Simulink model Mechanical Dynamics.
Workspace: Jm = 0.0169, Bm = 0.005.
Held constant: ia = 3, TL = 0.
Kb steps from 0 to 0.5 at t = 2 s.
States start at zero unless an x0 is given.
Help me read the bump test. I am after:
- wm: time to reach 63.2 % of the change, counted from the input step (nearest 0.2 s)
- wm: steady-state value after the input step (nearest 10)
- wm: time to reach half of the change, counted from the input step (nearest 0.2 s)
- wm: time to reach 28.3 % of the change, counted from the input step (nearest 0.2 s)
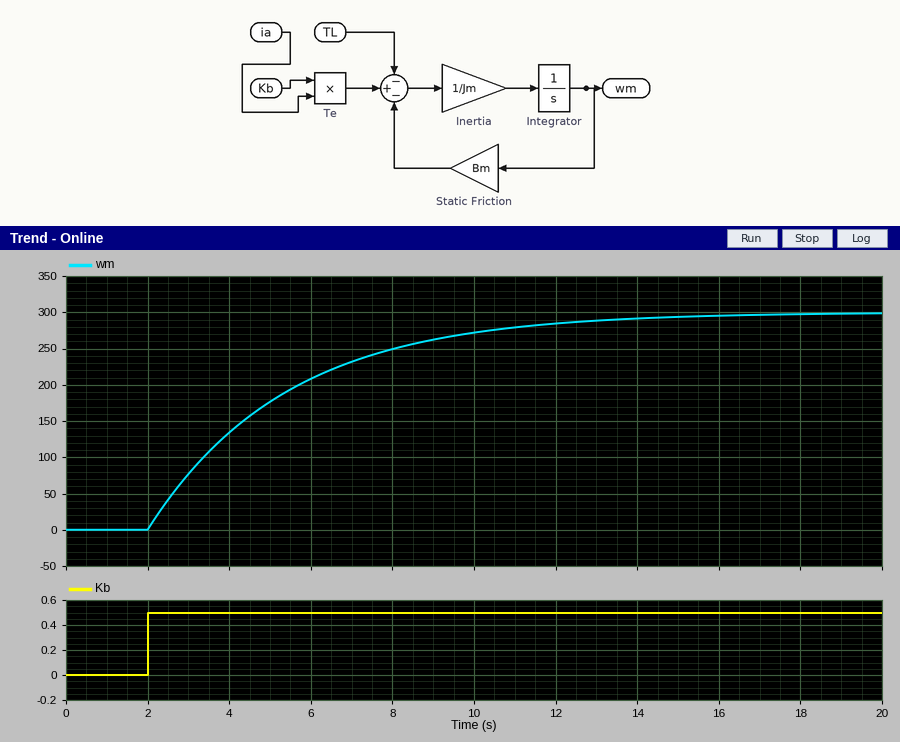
3.4 s
300
2.4 s
1.2 s
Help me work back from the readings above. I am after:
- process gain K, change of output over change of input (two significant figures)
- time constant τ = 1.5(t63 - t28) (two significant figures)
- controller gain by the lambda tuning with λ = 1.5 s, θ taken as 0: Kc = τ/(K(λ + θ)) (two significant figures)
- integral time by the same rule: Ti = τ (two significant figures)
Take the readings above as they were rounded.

600
3.3 s
0.0037
3.3 s
